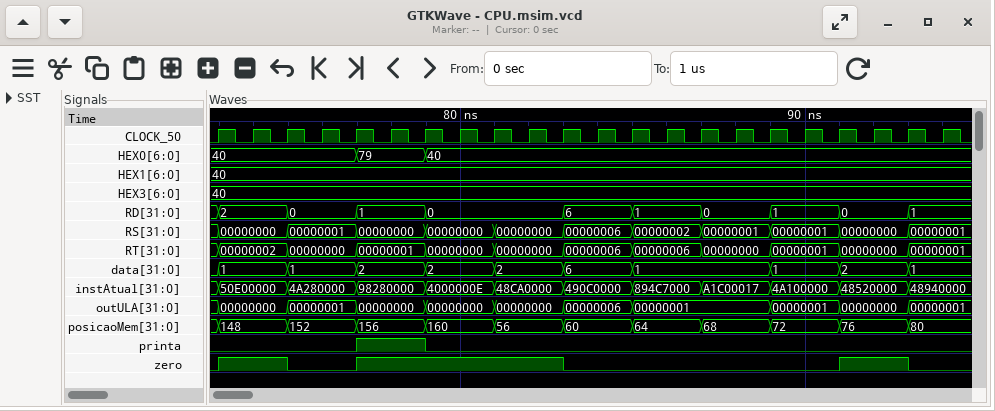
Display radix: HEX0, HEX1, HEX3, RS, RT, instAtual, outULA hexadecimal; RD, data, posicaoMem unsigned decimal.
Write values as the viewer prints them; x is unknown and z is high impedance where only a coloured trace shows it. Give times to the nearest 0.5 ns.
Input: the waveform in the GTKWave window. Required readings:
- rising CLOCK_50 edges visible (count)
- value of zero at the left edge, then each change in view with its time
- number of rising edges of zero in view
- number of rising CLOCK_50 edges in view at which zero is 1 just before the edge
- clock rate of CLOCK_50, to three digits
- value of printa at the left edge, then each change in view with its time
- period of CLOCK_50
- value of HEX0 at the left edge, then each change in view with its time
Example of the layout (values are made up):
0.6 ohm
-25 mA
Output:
22
0, 1 at 73 ns, 0 at 75 ns, 1 at 77 ns, 0 at 83 ns, 1 at 91 ns, 0 at 93 ns
3
10
1.00 GHz
0, 1 at 77 ns, 0 at 79 ns
1 ns
40, 79 at 77 ns, 40 at 79 ns
